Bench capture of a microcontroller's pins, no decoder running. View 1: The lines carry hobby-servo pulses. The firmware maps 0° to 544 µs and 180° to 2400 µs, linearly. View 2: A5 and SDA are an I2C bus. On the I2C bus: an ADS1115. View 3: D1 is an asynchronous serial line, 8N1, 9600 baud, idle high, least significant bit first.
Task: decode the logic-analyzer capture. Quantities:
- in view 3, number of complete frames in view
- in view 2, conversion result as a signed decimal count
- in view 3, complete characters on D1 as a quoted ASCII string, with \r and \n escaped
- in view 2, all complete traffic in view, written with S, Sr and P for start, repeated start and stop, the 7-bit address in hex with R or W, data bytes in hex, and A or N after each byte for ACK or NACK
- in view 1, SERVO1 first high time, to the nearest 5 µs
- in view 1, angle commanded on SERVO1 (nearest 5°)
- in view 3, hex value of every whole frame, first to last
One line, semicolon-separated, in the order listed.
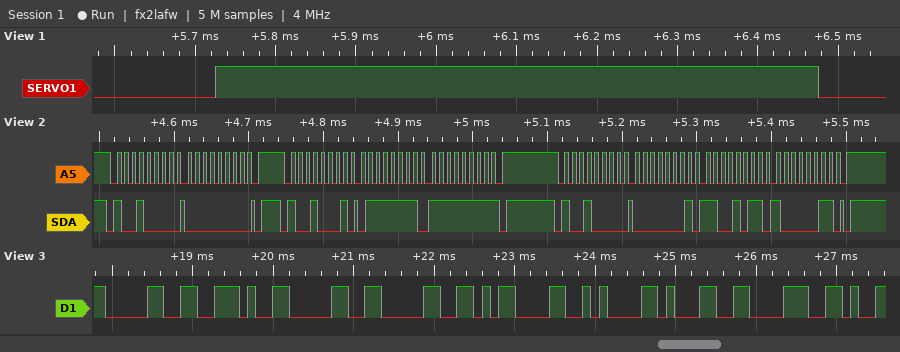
8; 32767; "0.00\r\n18"; S 48W A 00 A P S 48R A 7F A FF N P S 48W A 01 A CB A 83 A P; 750 µs; 20°; 30 2E 30 30 0D 0A 31 38
